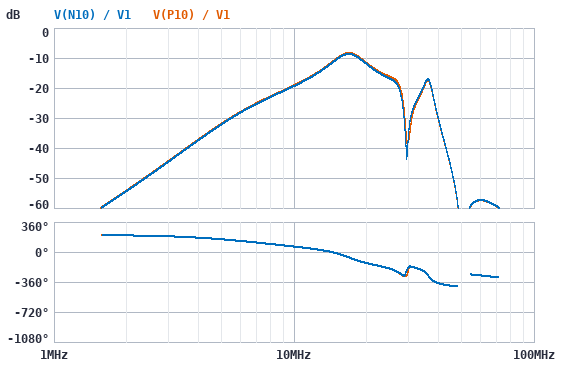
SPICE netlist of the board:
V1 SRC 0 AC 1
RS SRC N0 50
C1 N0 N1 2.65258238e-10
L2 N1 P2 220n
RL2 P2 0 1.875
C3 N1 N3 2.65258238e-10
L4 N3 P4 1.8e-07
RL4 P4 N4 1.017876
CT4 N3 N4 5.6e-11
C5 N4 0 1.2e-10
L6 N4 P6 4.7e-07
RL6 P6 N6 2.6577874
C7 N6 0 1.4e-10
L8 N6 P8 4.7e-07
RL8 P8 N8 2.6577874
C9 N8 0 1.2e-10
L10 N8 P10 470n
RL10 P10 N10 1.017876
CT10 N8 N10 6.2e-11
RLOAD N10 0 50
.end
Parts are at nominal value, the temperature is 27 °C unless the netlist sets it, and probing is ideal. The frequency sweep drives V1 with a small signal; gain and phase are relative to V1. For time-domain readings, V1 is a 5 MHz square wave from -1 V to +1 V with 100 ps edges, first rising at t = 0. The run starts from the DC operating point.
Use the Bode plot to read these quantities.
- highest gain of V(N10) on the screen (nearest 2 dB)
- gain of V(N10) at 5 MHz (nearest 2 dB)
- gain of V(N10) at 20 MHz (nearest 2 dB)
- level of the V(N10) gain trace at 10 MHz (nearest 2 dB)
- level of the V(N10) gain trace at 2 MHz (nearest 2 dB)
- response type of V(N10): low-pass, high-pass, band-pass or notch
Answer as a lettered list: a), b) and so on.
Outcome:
a) -8 dB
b) -32 dB
c) -12 dB
d) -20 dB
e) -54 dB
f) band-pass
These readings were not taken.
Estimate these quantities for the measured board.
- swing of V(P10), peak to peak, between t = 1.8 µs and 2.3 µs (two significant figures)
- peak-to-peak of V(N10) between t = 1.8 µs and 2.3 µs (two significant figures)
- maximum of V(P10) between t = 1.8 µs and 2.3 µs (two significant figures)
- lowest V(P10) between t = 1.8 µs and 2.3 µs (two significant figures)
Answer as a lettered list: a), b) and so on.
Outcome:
a) 360 mV
b) 350 mV
c) 180 mV
d) -180 mV
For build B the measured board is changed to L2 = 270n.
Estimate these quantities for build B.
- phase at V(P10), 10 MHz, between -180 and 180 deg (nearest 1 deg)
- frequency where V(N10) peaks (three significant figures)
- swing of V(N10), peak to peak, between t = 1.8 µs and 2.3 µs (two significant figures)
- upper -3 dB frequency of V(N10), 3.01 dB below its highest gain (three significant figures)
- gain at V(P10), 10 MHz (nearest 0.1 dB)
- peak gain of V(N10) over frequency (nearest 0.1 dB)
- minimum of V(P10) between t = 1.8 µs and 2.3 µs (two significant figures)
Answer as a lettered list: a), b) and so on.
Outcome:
a) 63 deg
b) 16.5 MHz
c) 420 mV
d) 19.9 MHz
e) -17.0 dB
f) -7.9 dB
g) -220 mV
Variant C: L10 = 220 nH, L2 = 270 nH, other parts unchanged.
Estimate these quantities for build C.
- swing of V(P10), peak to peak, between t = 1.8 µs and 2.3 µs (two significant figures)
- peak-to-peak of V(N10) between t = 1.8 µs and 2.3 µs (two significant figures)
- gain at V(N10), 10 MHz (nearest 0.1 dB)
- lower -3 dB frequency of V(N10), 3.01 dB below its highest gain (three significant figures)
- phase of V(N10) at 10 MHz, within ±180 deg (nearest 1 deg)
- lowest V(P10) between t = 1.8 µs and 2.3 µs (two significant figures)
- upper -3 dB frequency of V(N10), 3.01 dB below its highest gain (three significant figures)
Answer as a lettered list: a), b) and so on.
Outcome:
a) 660 mV
b) 640 mV
c) -16.0 dB
d) 14.2 MHz
e) 71 deg
f) -330 mV
g) 33.8 MHz
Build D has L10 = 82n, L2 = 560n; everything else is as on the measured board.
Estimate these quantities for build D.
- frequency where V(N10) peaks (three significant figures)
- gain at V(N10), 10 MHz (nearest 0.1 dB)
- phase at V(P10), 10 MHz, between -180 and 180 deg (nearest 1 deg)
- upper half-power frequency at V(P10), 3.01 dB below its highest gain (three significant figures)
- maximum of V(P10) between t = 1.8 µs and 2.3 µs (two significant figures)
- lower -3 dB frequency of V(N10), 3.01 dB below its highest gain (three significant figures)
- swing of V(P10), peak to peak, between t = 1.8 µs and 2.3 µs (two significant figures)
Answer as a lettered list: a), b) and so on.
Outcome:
a) 17.4 MHz
b) -8.6 dB
c) 46 deg
d) 37.0 MHz
e) 400 mV
f) 8.95 MHz
g) 800 mV
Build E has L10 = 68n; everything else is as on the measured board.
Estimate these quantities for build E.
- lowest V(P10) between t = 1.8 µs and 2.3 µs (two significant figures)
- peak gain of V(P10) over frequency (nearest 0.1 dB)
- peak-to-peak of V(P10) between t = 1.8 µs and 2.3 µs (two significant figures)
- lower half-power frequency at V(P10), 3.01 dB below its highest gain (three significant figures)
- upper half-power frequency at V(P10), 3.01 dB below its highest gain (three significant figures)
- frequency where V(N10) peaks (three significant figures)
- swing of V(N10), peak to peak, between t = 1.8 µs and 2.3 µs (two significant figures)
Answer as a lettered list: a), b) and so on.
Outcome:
a) -310 mV
b) -7.4 dB
c) 620 mV
d) 17.2 MHz
e) 37.1 MHz
f) 25.1 MHz
g) 610 mV
